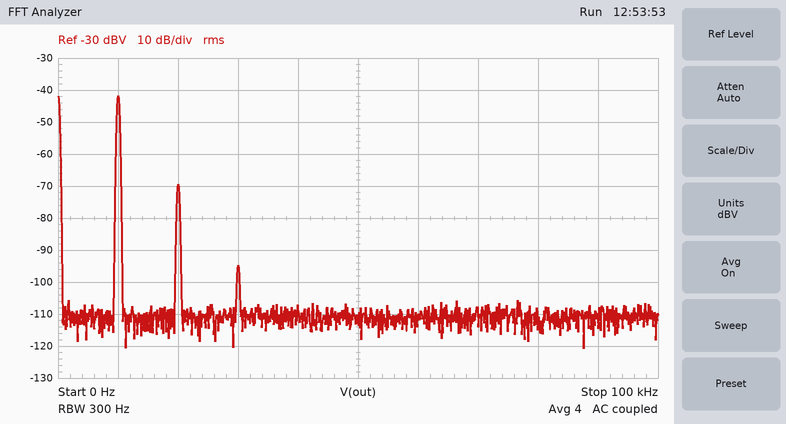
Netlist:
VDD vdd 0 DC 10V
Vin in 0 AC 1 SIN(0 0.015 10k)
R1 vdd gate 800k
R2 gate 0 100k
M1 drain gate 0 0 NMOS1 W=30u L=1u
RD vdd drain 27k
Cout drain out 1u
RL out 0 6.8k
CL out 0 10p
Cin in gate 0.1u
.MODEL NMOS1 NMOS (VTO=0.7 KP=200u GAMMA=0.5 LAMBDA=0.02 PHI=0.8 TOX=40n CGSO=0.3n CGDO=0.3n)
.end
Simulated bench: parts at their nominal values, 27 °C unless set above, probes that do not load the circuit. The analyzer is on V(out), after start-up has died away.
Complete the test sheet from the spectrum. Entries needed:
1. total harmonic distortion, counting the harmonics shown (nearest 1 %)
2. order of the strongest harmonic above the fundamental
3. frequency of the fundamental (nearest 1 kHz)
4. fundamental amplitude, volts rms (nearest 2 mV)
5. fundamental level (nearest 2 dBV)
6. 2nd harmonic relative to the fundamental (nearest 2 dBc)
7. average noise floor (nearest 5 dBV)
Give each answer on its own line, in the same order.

4 %
2
10 kHz
8 mV
-42 dBV
-28 dBc
-110 dBV
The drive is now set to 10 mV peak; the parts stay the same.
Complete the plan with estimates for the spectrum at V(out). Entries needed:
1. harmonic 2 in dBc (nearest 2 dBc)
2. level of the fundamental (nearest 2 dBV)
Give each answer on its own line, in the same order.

-32 dBc
-46 dBV
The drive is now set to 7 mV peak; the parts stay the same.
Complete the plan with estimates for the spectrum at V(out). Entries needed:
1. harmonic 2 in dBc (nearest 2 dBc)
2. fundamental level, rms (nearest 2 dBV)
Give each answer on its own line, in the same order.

-34 dBc
-48 dBV
